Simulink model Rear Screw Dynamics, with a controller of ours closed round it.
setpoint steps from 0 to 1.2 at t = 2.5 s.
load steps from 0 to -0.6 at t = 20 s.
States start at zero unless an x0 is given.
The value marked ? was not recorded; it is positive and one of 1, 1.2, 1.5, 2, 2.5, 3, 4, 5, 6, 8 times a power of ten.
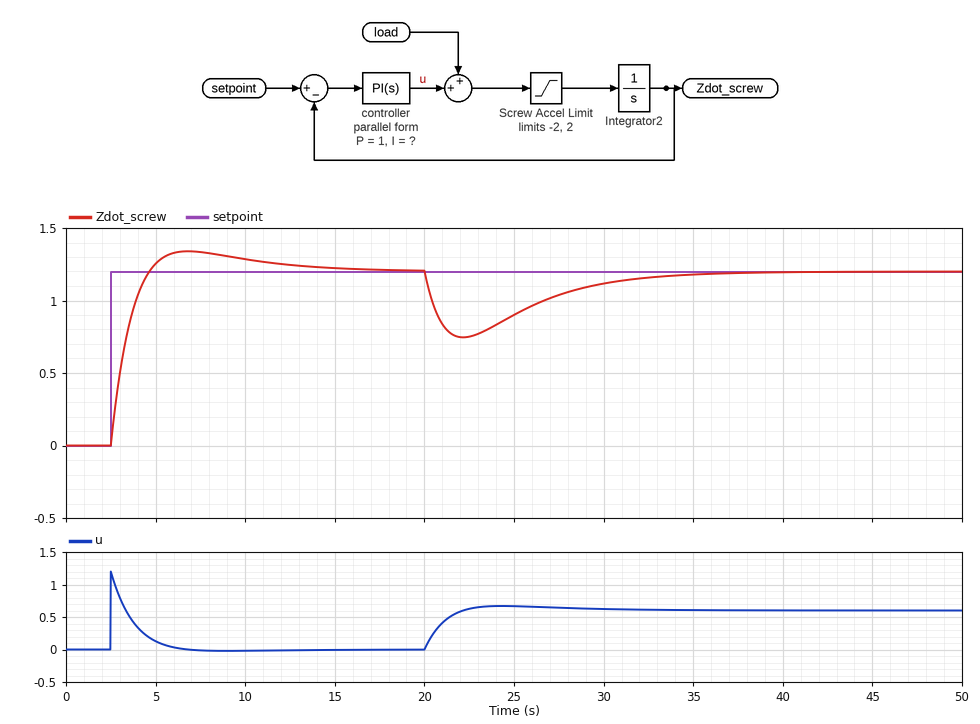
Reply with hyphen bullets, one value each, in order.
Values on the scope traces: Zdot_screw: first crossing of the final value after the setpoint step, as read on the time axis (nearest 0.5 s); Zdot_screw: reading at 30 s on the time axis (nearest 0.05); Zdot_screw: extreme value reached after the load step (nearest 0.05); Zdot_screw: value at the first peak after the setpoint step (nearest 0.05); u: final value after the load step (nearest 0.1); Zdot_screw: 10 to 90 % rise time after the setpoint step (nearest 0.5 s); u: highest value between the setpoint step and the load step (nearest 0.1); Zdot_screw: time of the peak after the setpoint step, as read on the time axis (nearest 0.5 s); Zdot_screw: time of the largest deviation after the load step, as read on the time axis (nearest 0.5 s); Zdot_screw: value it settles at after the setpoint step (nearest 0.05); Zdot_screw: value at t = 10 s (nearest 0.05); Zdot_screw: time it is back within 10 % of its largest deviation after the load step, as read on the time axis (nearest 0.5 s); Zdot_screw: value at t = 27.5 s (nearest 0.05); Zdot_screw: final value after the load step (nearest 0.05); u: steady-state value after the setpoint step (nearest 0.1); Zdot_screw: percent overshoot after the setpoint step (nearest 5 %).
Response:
- 4.5 s
- 1.10
- 0.75
- 1.35
- 0.6
- 1.5 s
- 1.2
- 7.0 s
- 22.0 s
- 1.20
- 1.30
- 32.0 s
- 1.05
- 1.20
- 0.0
- 10 %
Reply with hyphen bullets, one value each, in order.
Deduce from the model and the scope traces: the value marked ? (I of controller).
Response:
- 0.2
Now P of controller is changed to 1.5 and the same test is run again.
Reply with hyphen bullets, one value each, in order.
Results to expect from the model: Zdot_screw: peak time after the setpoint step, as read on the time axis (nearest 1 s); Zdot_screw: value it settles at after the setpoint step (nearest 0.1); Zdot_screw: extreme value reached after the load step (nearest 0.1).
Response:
- 6 s
- 1.2
- 0.9
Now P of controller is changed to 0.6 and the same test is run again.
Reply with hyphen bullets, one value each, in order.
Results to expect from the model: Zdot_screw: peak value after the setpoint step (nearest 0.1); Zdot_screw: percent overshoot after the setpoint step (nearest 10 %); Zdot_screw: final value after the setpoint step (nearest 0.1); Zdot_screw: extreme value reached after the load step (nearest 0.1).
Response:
- 1.5
- 20 %
- 1.2
- 0.6
